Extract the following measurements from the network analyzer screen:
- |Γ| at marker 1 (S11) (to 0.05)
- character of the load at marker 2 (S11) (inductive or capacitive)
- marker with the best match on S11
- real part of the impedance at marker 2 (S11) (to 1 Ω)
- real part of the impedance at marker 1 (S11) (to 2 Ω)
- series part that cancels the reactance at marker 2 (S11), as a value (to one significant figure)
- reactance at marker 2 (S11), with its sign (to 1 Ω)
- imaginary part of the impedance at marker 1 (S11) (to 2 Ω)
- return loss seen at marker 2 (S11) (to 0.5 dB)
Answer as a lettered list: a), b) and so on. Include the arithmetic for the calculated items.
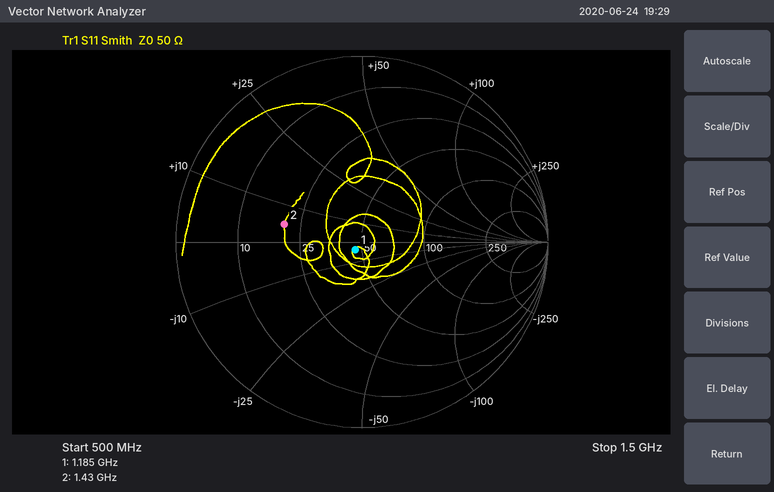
a) 0.05
b) inductive
c) marker 1
d) 20 Ω
e) 46 Ω
f) C = 1/(2π × 1.43 GHz × 5 Ω) ≈ 22.3 pF, so 20 pF to one significant figure
g) +5 Ω
h) -4 Ω
i) 7.5 dB
